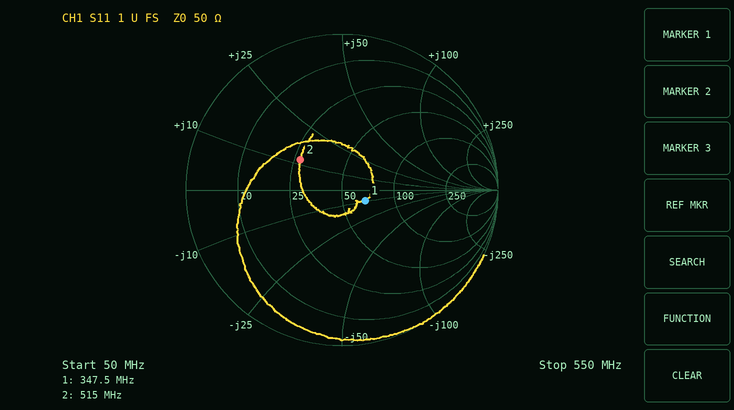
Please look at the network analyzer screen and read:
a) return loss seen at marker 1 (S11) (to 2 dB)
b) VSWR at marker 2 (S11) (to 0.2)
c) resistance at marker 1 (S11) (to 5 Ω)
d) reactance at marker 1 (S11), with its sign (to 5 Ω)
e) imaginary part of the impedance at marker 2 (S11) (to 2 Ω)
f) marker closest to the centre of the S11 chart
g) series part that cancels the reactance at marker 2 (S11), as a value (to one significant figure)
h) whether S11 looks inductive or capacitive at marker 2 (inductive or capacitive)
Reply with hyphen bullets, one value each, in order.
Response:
- 16 dB
- 2.0
- 65 Ω
- -10 Ω
- +12 Ω
- marker 1
- 30 pF
- inductive
